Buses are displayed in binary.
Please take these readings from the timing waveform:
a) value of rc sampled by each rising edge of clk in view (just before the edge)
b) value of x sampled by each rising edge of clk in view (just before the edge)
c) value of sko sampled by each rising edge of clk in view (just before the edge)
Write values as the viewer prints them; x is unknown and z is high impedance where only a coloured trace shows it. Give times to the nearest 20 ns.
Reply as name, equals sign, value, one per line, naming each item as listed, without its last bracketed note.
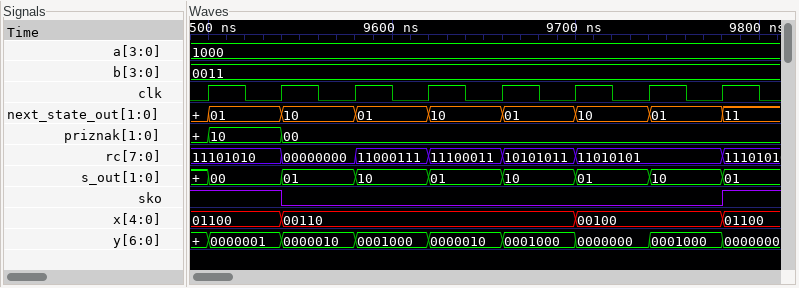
value of rc sampled by each rising edge of clk in view = 11101010, 11101010, 00000000, 11000111, 11100011, 10101011, 11010101, 11010101
value of x sampled by each rising edge of clk in view = 01100, 01100, 00110, 00110, 00110, 00110, 00100, 00100
value of sko sampled by each rising edge of clk in view = 1 1 0 0 0 0 0 0
